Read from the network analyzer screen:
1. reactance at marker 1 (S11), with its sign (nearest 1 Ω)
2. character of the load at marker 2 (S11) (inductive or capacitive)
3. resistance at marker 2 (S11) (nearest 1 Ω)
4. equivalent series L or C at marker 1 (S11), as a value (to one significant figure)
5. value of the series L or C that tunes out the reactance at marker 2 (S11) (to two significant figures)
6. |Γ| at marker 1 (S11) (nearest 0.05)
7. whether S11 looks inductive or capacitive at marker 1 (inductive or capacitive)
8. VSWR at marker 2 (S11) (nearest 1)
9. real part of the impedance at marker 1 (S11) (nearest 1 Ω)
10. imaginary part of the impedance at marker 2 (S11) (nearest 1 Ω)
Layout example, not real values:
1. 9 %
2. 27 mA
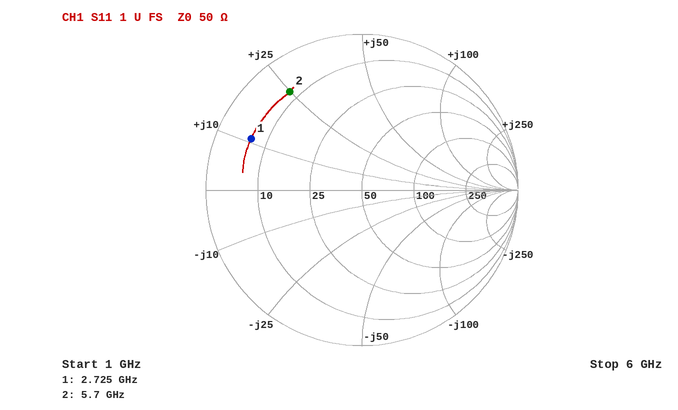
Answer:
1. +11 Ω
2. inductive
3. 8 Ω
4. 600 pH
5. 1.1 pF
6. 0.80
7. inductive
8. 8
9. 6 Ω
10. +25 Ω
